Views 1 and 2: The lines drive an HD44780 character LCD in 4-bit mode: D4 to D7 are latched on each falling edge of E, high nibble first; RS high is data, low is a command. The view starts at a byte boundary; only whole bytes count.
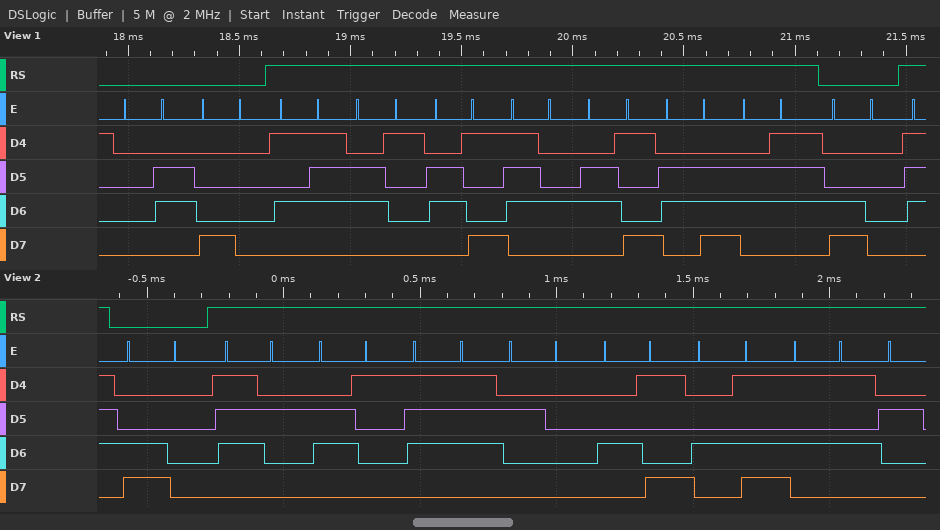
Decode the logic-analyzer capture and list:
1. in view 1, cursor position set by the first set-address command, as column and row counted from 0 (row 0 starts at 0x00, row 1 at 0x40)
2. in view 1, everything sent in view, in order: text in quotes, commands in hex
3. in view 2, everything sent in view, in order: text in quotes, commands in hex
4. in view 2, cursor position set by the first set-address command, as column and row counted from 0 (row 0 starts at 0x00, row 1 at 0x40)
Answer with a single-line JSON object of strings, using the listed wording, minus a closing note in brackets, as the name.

{"in view 1, cursor position set by the first set-address command, as column and row counted from 0": "column 0, row 0", "in view 1, everything sent in view, in order: text in quotes, commands in hex": "0x06 0x80 \"Waiting\" 0xC0", "in view 2, everything sent in view, in order: text in quotes, commands in hex": "0xC0 \"raw IMU\"", "in view 2, cursor position set by the first set-address command, as column and row counted from 0": "column 0, row 1"}
